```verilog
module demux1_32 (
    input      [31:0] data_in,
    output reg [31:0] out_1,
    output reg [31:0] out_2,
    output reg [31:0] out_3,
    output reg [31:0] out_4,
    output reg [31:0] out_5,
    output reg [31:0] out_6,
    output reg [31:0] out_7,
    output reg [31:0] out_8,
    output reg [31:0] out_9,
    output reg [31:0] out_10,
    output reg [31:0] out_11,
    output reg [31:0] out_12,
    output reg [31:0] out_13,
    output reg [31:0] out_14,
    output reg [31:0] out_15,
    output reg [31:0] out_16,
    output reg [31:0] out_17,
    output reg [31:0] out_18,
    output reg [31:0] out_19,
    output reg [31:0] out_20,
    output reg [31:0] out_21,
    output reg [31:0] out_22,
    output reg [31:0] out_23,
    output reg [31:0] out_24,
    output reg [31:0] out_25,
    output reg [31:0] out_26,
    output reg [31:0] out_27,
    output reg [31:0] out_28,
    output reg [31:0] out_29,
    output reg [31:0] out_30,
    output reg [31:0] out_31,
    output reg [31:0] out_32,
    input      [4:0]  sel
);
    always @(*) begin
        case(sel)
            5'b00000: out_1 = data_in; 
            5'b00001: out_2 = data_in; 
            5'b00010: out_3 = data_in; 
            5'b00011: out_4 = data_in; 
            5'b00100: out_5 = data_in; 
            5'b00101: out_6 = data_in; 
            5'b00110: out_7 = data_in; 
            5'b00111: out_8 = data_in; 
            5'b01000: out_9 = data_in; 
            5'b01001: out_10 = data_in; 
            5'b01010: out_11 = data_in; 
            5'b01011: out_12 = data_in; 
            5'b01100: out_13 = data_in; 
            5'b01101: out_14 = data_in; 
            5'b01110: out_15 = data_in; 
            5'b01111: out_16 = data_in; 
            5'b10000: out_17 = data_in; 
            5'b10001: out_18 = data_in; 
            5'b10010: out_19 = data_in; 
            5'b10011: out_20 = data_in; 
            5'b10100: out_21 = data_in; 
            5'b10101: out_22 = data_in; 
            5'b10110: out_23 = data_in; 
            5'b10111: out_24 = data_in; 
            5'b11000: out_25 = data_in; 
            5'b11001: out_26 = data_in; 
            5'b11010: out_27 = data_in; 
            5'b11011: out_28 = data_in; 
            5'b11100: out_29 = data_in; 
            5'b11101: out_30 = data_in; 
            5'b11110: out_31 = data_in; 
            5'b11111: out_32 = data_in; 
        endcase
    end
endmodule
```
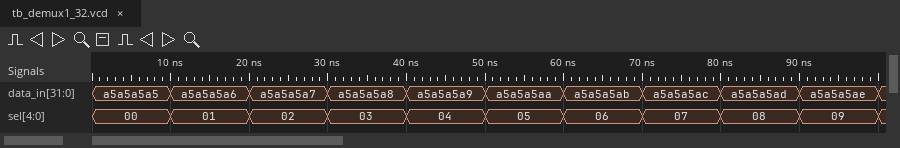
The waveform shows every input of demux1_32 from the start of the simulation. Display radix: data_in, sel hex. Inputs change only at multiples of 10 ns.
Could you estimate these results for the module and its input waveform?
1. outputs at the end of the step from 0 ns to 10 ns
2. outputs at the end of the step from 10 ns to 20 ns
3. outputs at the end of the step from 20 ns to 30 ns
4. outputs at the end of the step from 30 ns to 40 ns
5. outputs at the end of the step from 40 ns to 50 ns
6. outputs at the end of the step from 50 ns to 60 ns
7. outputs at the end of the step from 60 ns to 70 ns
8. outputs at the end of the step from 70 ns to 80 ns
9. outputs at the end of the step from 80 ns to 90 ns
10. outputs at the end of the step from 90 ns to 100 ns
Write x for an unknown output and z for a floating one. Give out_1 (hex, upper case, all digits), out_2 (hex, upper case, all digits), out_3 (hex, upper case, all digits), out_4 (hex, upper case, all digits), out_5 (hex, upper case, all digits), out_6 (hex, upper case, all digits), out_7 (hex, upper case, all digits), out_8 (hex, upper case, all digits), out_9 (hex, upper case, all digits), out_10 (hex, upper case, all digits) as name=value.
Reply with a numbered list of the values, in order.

1. out_1=A5A5A5A5, out_2=x, out_3=x, out_4=x, out_5=x, out_6=x, out_7=x, out_8=x, out_9=x, out_10=x
2. out_1=A5A5A5A5, out_2=A5A5A5A6, out_3=x, out_4=x, out_5=x, out_6=x, out_7=x, out_8=x, out_9=x, out_10=x
3. out_1=A5A5A5A5, out_2=A5A5A5A6, out_3=A5A5A5A7, out_4=x, out_5=x, out_6=x, out_7=x, out_8=x, out_9=x, out_10=x
4. out_1=A5A5A5A5, out_2=A5A5A5A6, out_3=A5A5A5A7, out_4=A5A5A5A8, out_5=x, out_6=x, out_7=x, out_8=x, out_9=x, out_10=x
5. out_1=A5A5A5A5, out_2=A5A5A5A6, out_3=A5A5A5A7, out_4=A5A5A5A8, out_5=A5A5A5A9, out_6=x, out_7=x, out_8=x, out_9=x, out_10=x
6. out_1=A5A5A5A5, out_2=A5A5A5A6, out_3=A5A5A5A7, out_4=A5A5A5A8, out_5=A5A5A5A9, out_6=A5A5A5AA, out_7=x, out_8=x, out_9=x, out_10=x
7. out_1=A5A5A5A5, out_2=A5A5A5A6, out_3=A5A5A5A7, out_4=A5A5A5A8, out_5=A5A5A5A9, out_6=A5A5A5AA, out_7=A5A5A5AB, out_8=x, out_9=x, out_10=x
8. out_1=A5A5A5A5, out_2=A5A5A5A6, out_3=A5A5A5A7, out_4=A5A5A5A8, out_5=A5A5A5A9, out_6=A5A5A5AA, out_7=A5A5A5AB, out_8=A5A5A5AC, out_9=x, out_10=x
9. out_1=A5A5A5A5, out_2=A5A5A5A6, out_3=A5A5A5A7, out_4=A5A5A5A8, out_5=A5A5A5A9, out_6=A5A5A5AA, out_7=A5A5A5AB, out_8=A5A5A5AC, out_9=A5A5A5AD, out_10=x
10. out_1=A5A5A5A5, out_2=A5A5A5A6, out_3=A5A5A5A7, out_4=A5A5A5A8, out_5=A5A5A5A9, out_6=A5A5A5AA, out_7=A5A5A5AB, out_8=A5A5A5AC, out_9=A5A5A5AD, out_10=A5A5A5AE
